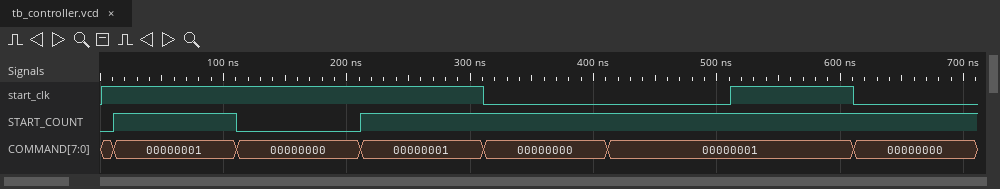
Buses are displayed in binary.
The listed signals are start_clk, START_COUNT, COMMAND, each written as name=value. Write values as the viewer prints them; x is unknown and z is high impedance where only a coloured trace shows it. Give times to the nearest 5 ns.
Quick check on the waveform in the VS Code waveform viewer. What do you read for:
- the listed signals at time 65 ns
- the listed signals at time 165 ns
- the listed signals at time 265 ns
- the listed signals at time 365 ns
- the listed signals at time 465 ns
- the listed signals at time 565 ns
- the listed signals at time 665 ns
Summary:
start_clk=1, START_COUNT=1, COMMAND=00000001
start_clk=1, START_COUNT=0, COMMAND=00000000
start_clk=1, START_COUNT=1, COMMAND=00000001
start_clk=0, START_COUNT=1, COMMAND=00000000
start_clk=0, START_COUNT=1, COMMAND=00000001
start_clk=1, START_COUNT=1, COMMAND=00000001
start_clk=0, START_COUNT=1, COMMAND=00000000
